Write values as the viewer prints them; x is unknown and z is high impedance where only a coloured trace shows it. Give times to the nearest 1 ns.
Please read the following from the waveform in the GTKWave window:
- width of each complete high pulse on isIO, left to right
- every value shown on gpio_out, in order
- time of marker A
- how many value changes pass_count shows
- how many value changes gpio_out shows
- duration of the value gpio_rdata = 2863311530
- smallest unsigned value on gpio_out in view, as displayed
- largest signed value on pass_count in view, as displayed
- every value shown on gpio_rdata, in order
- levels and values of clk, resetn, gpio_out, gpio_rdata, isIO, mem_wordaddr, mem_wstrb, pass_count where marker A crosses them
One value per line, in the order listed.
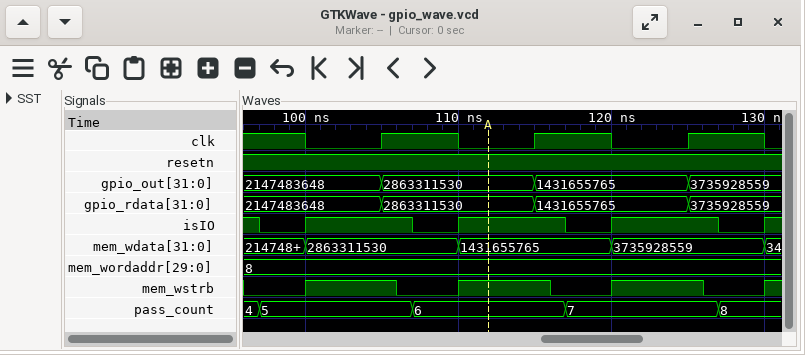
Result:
7 ns, 7 ns, 7 ns
2147483648, 2863311530, 1431655765, 3735928559
112 ns
4
3
10 ns
1431655765
8
2147483648, 2863311530, 1431655765, 3735928559
clk=0, resetn=1, gpio_out=2863311530, gpio_rdata=2863311530, isIO=1, mem_wordaddr=8, mem_wstrb=1, pass_count=6
